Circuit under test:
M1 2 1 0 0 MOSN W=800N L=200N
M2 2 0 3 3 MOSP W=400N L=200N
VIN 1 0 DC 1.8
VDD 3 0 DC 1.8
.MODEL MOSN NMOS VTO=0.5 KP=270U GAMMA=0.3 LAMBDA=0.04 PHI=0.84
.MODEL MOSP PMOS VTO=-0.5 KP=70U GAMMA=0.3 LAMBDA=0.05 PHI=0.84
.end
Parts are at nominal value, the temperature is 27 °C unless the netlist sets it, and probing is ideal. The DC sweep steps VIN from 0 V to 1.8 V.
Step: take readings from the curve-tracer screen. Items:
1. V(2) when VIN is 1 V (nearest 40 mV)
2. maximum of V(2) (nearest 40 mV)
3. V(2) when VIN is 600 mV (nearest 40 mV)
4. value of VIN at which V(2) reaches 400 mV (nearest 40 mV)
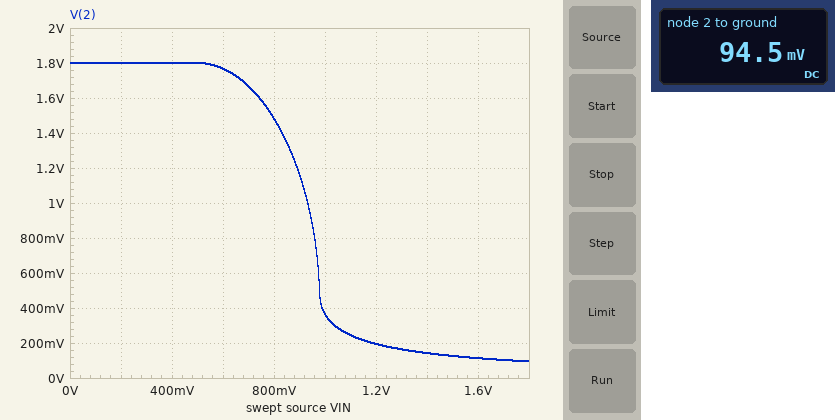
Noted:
360 mV
1.80 V
1.76 V
1.00 V
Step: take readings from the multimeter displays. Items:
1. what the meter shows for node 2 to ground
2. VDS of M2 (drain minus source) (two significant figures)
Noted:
94.5 mV
-1.7 V
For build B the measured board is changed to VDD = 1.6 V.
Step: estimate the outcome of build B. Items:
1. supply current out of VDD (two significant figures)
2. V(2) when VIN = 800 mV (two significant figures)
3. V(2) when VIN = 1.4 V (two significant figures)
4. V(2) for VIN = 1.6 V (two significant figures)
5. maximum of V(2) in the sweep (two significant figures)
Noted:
91 µA
1.2 V
99 mV
79 mV
1.6 V
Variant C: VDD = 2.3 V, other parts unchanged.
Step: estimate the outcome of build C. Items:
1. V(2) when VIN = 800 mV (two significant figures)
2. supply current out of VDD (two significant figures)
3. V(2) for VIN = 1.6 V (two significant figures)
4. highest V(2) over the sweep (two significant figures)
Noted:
2.1 V
250 µA
230 mV
2.3 V
